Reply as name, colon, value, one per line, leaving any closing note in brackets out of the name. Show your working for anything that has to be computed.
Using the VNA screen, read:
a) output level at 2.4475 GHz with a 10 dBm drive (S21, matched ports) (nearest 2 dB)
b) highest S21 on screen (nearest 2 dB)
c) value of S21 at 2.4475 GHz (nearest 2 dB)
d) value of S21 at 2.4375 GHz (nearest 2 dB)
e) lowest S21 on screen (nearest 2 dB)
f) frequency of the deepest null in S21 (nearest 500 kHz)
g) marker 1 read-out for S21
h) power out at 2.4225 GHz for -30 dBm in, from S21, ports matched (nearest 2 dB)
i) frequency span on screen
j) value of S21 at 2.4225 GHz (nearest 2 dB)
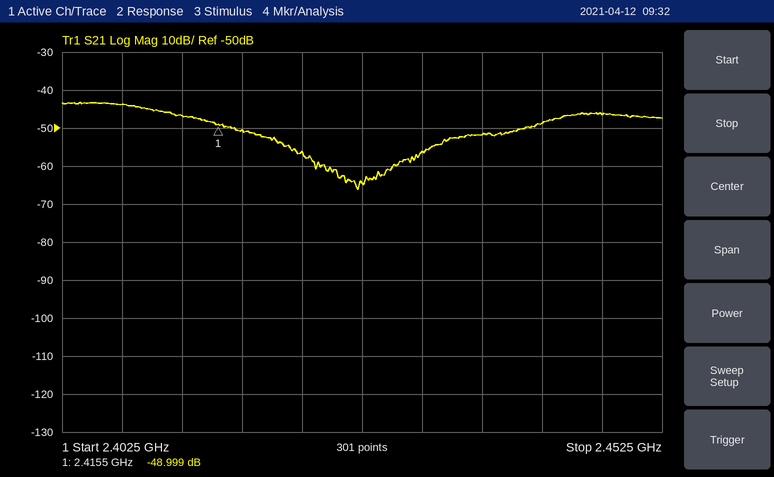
output level at 2.4475 GHz with a 10 dBm drive (S21, matched ports): 10 dBm + (-46 dB) = -36 dBm
highest S21 on screen: -44 dB
value of S21 at 2.4475 GHz: -46 dB
value of S21 at 2.4375 GHz: -52 dB
lowest S21 on screen: -66 dB
frequency of the deepest null in S21: 2.4270 GHz
marker 1 read-out for S21: -48.999 dB
power out at 2.4225 GHz for -30 dBm in, from S21, ports matched: -30 dBm + (-56 dB) = -86 dBm
frequency span on screen: 50 MHz
value of S21 at 2.4225 GHz: -56 dB
